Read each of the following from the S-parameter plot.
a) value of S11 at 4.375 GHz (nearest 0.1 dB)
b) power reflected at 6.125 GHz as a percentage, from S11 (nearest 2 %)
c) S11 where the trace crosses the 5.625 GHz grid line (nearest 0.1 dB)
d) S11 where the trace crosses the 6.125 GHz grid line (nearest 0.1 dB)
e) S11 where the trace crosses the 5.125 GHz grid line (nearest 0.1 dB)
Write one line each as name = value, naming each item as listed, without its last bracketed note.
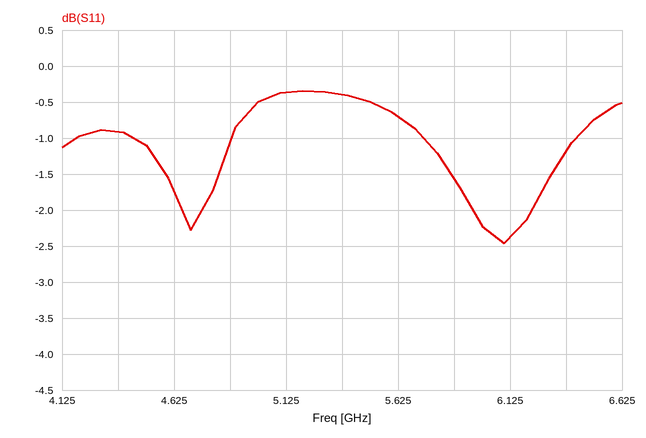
value of S11 at 4.375 GHz = -0.9 dB
power reflected at 6.125 GHz as a percentage, from S11 = 58 %
S11 where the trace crosses the 5.625 GHz grid line = -0.7 dB
S11 where the trace crosses the 6.125 GHz grid line = -2.4 dB
S11 where the trace crosses the 5.125 GHz grid line = -0.4 dB
